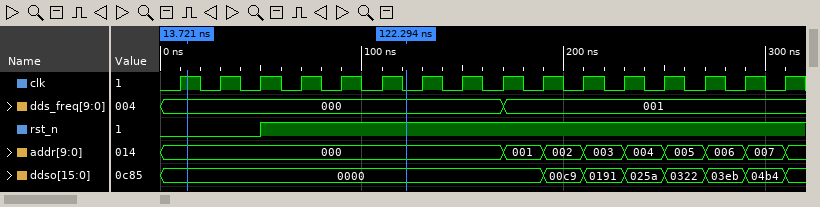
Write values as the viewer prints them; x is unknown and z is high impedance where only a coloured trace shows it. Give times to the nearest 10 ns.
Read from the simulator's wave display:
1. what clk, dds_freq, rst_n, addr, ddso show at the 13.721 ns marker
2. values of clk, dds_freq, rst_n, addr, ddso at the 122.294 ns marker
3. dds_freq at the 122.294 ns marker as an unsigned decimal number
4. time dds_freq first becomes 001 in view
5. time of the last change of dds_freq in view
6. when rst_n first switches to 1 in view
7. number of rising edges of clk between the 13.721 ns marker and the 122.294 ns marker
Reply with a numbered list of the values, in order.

1. clk=1, dds_freq=000, rst_n=0, addr=000, ddso=0000
2. clk=0, dds_freq=000, rst_n=1, addr=000, ddso=0000
3. 0
4. 170 ns
5. 170 ns
6. 50 ns
7. 5
